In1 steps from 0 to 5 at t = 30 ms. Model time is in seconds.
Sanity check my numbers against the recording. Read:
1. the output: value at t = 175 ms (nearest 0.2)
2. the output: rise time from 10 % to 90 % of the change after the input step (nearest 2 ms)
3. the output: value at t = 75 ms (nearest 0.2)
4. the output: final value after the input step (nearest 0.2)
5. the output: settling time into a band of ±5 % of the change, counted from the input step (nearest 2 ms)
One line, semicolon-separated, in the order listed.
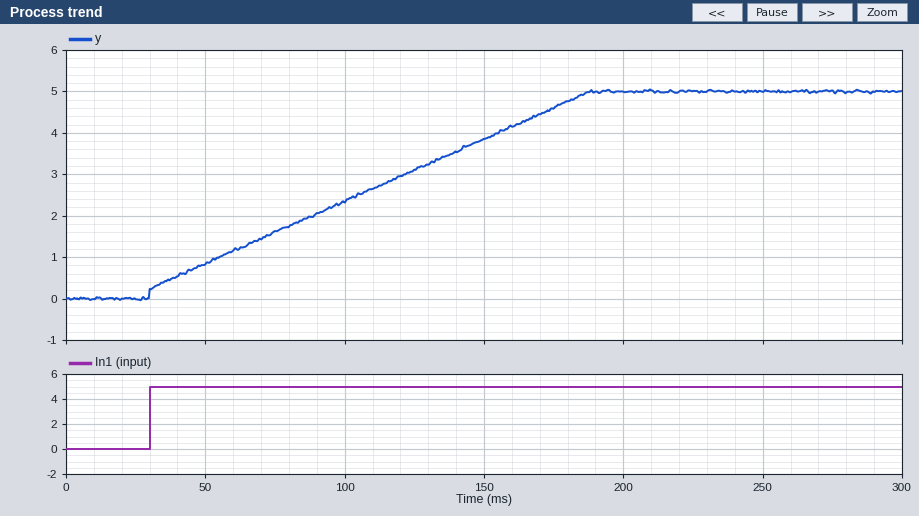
4.6; 134 ms; 1.6; 5.0; 150 ms
